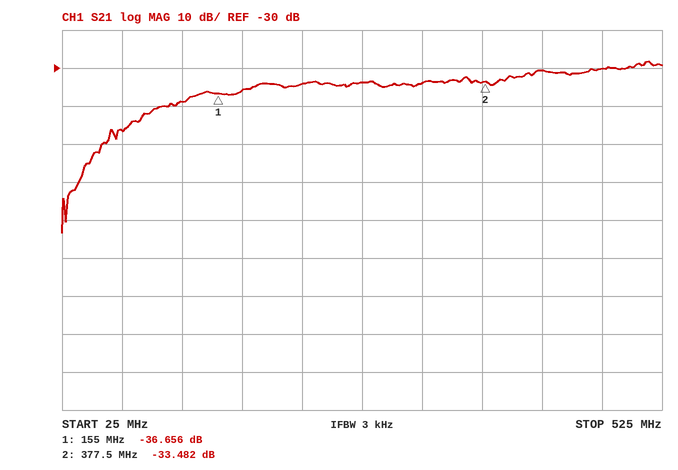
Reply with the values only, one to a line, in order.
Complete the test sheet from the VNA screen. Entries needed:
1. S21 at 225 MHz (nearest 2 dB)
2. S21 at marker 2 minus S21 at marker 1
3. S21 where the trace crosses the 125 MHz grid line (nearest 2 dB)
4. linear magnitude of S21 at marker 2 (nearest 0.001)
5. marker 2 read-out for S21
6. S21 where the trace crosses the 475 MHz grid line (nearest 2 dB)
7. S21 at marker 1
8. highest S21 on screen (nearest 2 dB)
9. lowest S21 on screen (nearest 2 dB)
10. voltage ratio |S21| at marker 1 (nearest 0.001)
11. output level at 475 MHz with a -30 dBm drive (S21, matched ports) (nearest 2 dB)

-34 dB
3.174 dB
-38 dB
0.021
-33.482 dB
-30 dB
-36.656 dB
-28 dB
-74 dB
0.015
-60 dBm
